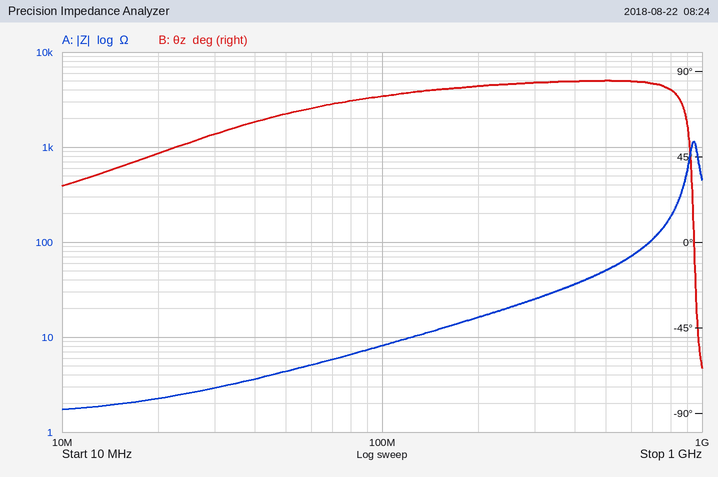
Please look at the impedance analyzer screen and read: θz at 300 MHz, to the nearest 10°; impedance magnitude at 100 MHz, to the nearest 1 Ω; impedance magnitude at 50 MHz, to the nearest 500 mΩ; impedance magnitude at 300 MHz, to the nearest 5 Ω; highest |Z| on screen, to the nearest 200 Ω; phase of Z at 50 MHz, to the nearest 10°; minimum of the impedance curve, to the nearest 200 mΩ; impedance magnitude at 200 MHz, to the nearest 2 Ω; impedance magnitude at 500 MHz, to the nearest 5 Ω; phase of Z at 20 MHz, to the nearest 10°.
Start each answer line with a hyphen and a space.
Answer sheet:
- 80°
- 8 Ω
- 4.5 Ω
- 25 Ω
- 1.2 kΩ
- 70°
- 1.8 Ω
- 16 Ω
- 50 Ω
- 50°
